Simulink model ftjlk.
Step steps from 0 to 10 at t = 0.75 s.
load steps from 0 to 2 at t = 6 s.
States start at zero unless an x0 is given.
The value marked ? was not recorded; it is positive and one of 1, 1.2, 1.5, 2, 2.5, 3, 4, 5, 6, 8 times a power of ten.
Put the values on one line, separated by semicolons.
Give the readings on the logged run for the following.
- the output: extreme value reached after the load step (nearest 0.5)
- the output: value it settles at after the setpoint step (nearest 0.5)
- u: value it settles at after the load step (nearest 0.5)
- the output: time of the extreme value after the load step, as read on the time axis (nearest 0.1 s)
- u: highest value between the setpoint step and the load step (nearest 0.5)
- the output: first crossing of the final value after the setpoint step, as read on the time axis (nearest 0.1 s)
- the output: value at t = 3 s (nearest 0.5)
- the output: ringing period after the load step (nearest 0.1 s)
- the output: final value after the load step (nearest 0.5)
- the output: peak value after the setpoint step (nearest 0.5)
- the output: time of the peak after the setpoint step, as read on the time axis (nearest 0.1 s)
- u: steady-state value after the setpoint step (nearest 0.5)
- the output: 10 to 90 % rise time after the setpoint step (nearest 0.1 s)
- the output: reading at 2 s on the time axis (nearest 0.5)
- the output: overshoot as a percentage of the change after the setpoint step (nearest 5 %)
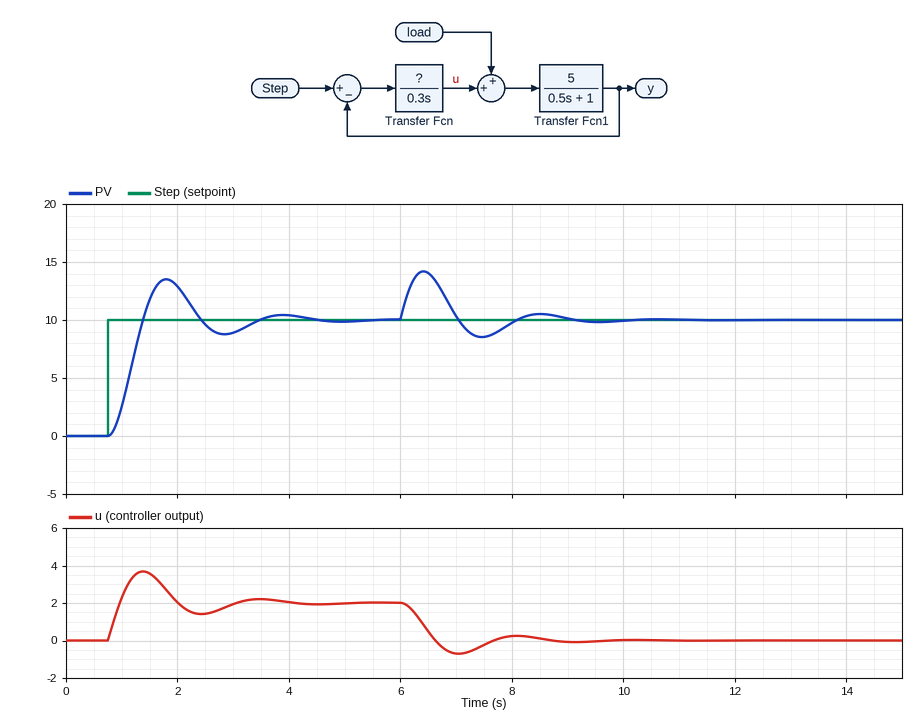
14.0; 10.0; 0.0; 6.4 s; 3.5; 1.4 s; 9.0; 2.1 s; 10.0; 13.5; 1.8 s; 2.0; 0.4 s; 13.0; 35 %
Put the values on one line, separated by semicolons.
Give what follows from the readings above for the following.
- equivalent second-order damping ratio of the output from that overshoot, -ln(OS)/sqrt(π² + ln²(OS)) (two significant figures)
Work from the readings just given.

0.32
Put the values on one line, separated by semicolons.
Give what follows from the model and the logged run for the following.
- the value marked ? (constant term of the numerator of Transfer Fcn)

0.3
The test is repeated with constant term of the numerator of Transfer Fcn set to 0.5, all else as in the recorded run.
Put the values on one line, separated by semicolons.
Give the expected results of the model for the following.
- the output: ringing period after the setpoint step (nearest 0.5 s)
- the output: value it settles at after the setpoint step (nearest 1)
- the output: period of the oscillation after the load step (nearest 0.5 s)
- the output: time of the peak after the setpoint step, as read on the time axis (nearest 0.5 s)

1.5 s; 10; 1.5 s; 1.5 s
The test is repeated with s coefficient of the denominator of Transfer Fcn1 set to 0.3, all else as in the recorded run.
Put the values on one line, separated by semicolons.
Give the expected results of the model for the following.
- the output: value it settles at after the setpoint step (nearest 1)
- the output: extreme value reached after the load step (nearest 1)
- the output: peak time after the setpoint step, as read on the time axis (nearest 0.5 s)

10; 15; 1.5 s
